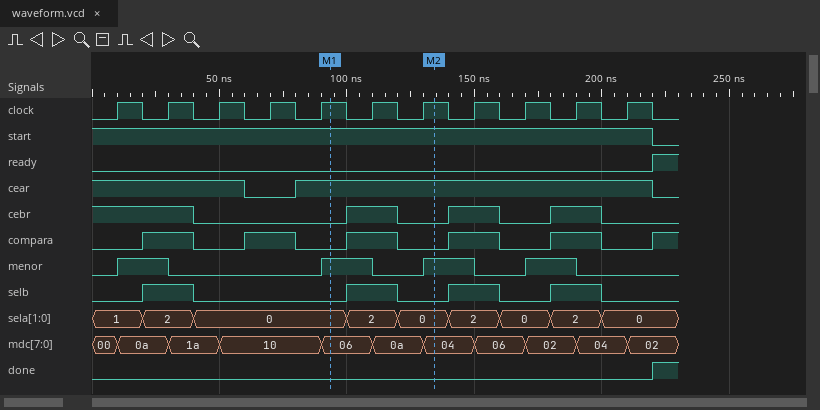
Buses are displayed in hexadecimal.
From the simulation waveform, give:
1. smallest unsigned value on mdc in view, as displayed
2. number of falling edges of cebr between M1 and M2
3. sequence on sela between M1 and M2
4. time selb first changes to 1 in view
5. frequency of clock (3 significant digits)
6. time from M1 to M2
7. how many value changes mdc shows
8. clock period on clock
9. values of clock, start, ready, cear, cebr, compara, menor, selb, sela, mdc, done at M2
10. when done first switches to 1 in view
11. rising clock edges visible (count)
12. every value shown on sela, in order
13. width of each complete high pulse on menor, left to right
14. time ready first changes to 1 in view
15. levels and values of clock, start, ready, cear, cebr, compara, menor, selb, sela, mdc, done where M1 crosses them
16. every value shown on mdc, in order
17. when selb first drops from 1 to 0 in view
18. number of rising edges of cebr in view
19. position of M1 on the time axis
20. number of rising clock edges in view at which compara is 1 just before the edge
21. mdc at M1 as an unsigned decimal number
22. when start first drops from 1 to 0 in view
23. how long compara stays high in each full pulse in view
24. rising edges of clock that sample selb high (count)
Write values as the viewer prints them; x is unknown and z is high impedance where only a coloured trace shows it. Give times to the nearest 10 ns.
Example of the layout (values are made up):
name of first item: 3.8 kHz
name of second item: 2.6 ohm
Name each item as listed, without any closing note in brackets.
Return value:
smallest unsigned value on mdc in view, as displayed: 00
number of falling edges of cebr between M1 and M2: 1
sequence on sela between M1 and M2: 0, 2, 0
time selb first changes to 1 in view: 20 ns
frequency of clock: 50.0 MHz
time from M1 to M2: 40 ns
how many value changes mdc shows: 10
clock period on clock: 20 ns
values of clock, start, ready, cear, cebr, compara, menor, selb, sela, mdc, done at M2: clock=1, start=1, ready=0, cear=1, cebr=0, compara=0, menor=1, selb=0, sela=0, mdc=04, done=0
when done first switches to 1 in view: 220 ns
rising clock edges visible: 11
every value shown on sela, in order: 1, 2, 0, 2, 0, 2, 0, 2, 0
width of each complete high pulse on menor, left to right: 20 ns, 20 ns, 20 ns, 20 ns
time ready first changes to 1 in view: 220 ns
levels and values of clock, start, ready, cear, cebr, compara, menor, selb, sela, mdc, done where M1 crosses them: clock=1, start=1, ready=0, cear=1, cebr=0, compara=0, menor=1, selb=0, sela=0, mdc=06, done=0
every value shown on mdc, in order: 00, 0a, 1a, 10, 06, 0a, 04, 06, 02, 04, 02
when selb first drops from 1 to 0 in view: 40 ns
number of rising edges of cebr in view: 3
position of M1 on the time axis: 90 ns
number of rising clock edges in view at which compara is 1 just before the edge: 5
mdc at M1 as an unsigned decimal number: 6
when start first drops from 1 to 0 in view: 220 ns
how long compara stays high in each full pulse in view: 20 ns, 20 ns, 20 ns, 20 ns, 20 ns
rising edges of clock that sample selb high: 4
